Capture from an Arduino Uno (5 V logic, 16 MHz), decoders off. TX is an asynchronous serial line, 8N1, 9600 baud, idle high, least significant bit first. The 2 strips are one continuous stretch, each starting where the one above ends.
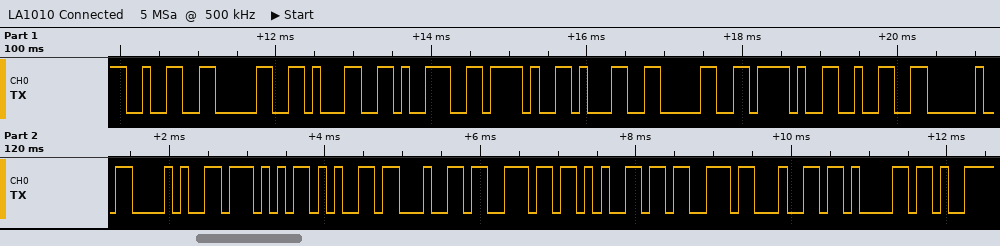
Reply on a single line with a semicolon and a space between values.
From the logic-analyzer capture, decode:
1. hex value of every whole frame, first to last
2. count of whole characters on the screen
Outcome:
32 30 31 39 2F 31 30 2F 32 20 28 57 65 64 6E 65 73 64 61; 19
